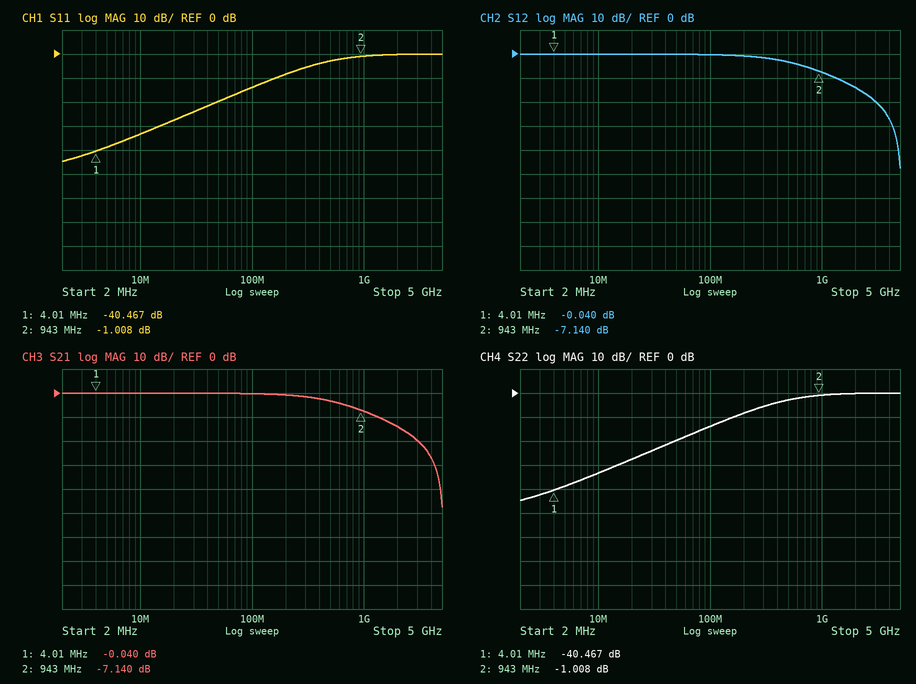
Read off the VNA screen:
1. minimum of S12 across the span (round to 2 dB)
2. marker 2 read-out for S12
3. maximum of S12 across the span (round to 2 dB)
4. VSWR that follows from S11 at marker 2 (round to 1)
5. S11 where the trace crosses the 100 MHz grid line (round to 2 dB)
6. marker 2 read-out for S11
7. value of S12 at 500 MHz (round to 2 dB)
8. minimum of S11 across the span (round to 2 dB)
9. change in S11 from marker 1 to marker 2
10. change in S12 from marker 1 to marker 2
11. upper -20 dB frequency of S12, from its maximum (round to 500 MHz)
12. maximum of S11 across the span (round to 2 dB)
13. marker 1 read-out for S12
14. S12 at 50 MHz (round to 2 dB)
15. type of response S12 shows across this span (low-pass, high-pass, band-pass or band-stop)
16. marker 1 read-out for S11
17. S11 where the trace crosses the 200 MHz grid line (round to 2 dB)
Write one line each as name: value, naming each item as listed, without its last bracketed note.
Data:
minimum of S12 across the span: -48 dB
marker 2 read-out for S12: -7.140 dB
maximum of S12 across the span: 0 dB
VSWR that follows from S11 at marker 2: 17
S11 where the trace crosses the 100 MHz grid line: -14 dB
marker 2 read-out for S11: -1.008 dB
value of S12 at 500 MHz: -4 dB
minimum of S11 across the span: -44 dB
change in S11 from marker 1 to marker 2: 39.459 dB
change in S12 from marker 1 to marker 2: -7.100 dB
upper -20 dB frequency of S12, from its maximum: 3.0 GHz
maximum of S11 across the span: 0 dB
marker 1 read-out for S12: -0.040 dB
S12 at 50 MHz: 0 dB
type of response S12 shows across this span: low-pass
marker 1 read-out for S11: -40.467 dB
S11 where the trace crosses the 200 MHz grid line: -8 dB
